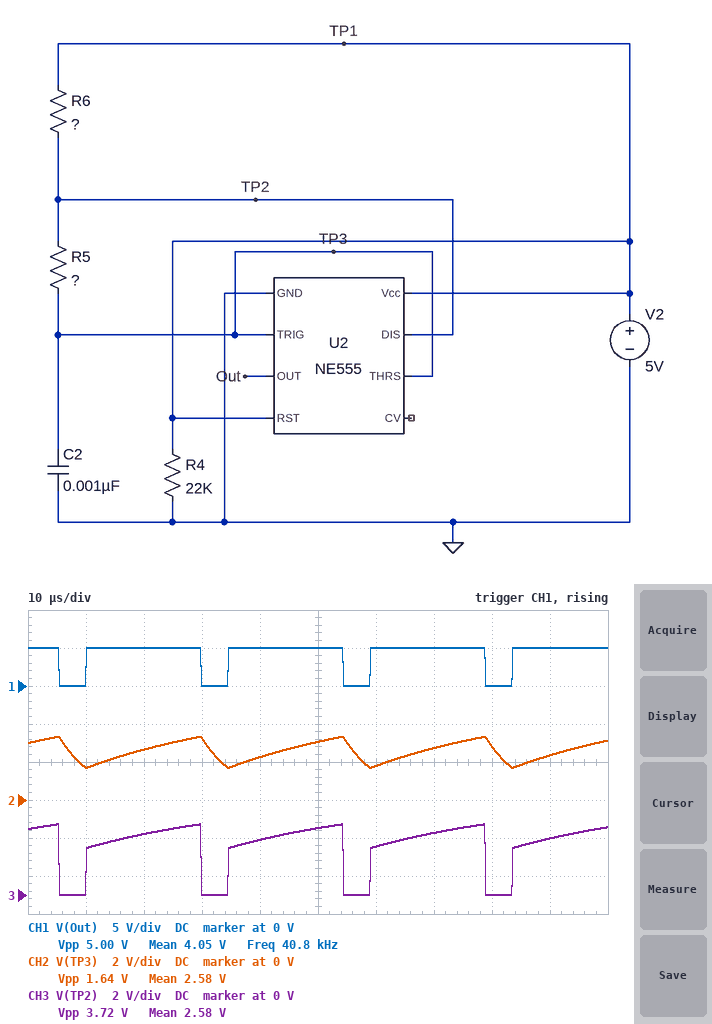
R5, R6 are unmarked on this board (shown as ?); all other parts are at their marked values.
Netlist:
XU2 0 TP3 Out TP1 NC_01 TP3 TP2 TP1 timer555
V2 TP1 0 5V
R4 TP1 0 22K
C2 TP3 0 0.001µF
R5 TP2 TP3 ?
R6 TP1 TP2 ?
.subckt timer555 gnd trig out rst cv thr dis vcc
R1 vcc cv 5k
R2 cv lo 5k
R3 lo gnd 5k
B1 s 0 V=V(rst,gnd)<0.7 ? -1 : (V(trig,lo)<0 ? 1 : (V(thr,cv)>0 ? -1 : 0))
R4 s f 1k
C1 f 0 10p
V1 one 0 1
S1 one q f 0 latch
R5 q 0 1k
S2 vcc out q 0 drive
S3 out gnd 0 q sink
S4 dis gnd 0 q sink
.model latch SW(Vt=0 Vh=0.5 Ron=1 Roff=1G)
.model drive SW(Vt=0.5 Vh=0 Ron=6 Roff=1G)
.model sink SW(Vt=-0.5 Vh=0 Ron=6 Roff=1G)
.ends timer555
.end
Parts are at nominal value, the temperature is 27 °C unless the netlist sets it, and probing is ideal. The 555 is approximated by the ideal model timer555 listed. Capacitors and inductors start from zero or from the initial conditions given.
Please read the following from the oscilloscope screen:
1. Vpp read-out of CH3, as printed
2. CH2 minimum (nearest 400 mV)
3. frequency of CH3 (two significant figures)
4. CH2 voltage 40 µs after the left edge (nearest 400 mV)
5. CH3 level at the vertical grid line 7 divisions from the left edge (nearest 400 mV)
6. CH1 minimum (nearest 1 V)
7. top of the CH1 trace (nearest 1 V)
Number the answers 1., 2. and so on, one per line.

1. 3.72 V
2. 1.6 V
3. 41 kHz
4. 2.4 V
5. 3.2 V
6. 0 V
7. 5 V
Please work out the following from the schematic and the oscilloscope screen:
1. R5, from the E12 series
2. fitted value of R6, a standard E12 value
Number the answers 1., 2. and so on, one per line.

1. 6.8 kΩ
2. 22 kΩ
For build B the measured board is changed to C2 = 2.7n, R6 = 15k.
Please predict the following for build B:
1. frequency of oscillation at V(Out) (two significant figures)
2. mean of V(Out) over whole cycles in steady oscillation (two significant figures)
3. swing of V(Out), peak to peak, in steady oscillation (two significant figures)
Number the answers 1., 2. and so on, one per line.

1. 19 kHz
2. 3.8 V
3. 5.0 V
